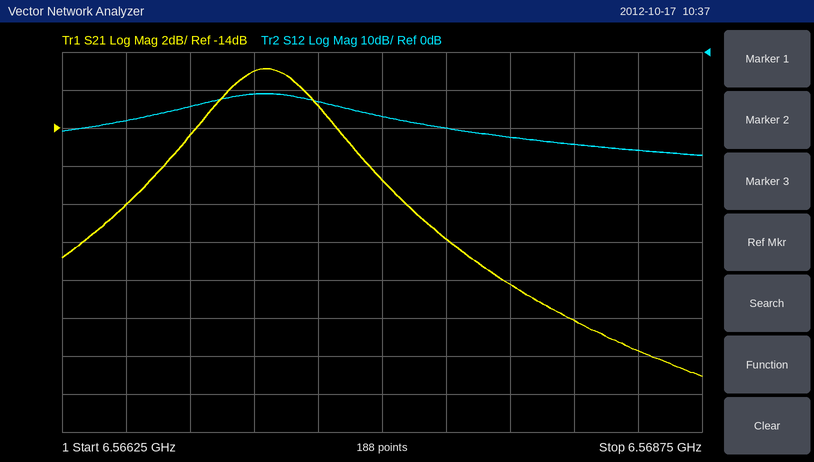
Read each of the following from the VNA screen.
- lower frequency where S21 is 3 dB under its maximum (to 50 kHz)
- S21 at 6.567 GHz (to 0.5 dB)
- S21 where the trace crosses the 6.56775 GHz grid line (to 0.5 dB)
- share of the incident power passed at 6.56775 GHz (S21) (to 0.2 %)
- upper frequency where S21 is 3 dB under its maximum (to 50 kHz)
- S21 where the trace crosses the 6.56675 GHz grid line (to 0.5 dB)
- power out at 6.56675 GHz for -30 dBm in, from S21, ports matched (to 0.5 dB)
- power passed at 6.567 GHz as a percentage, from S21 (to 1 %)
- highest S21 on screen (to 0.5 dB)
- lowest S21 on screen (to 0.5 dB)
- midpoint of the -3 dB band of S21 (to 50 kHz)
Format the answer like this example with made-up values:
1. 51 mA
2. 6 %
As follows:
1. 6.56680 GHz
2. -11.0 dB
3. -20.0 dB
4. 1.0 %
5. 6.56730 GHz
6. -14.5 dB
7. -44.5 dBm
8. 8 %
9. -11.0 dB
10. -27.0 dB
11. 6.56705 GHz
